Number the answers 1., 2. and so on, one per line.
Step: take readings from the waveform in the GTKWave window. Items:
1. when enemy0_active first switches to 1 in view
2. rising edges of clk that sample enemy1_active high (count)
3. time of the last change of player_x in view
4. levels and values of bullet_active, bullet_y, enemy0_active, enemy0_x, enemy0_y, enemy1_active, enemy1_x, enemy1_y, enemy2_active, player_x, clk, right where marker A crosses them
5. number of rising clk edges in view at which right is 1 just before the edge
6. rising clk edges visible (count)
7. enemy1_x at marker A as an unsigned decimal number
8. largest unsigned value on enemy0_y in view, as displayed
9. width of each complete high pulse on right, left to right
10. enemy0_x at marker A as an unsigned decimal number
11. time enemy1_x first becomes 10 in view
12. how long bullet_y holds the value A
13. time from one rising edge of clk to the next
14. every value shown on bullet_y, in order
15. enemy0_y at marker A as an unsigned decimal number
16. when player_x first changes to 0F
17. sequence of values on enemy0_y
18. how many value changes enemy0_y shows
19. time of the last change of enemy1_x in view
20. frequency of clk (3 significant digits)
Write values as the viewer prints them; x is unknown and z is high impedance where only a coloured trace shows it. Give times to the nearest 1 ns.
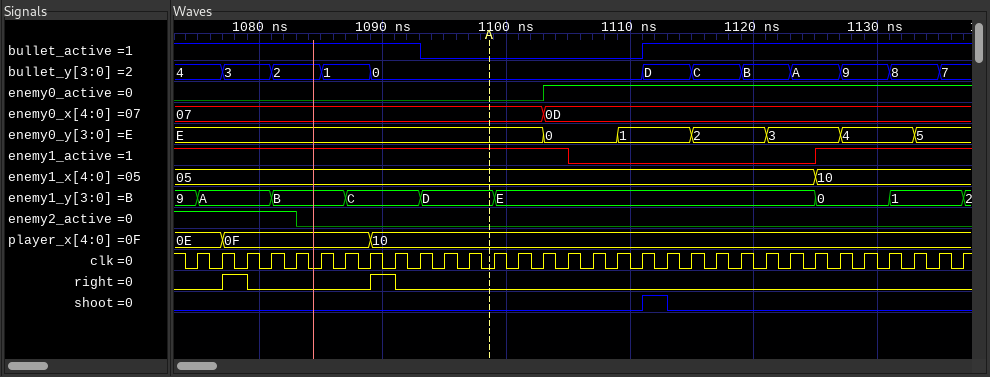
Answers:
1. 1103 ns
2. 22
3. 1089 ns
4. bullet_active=0, bullet_y=0, enemy0_active=0, enemy0_x=07, enemy0_y=E, enemy1_active=1, enemy1_x=05, enemy1_y=D, enemy2_active=0, player_x=10, clk=0, right=0
5. 2
6. 32
7. 5
8. E
9. 2 ns, 2 ns
10. 7
11. 1125 ns
12. 4 ns
13. 2 ns
14. 4, 3, 2, 1, 0, D, C, B, A, 9, 8, 7
15. 14
16. 1077 ns
17. E, 0, 1, 2, 3, 4, 5
18. 6
19. 1125 ns
20. 500 MHz
